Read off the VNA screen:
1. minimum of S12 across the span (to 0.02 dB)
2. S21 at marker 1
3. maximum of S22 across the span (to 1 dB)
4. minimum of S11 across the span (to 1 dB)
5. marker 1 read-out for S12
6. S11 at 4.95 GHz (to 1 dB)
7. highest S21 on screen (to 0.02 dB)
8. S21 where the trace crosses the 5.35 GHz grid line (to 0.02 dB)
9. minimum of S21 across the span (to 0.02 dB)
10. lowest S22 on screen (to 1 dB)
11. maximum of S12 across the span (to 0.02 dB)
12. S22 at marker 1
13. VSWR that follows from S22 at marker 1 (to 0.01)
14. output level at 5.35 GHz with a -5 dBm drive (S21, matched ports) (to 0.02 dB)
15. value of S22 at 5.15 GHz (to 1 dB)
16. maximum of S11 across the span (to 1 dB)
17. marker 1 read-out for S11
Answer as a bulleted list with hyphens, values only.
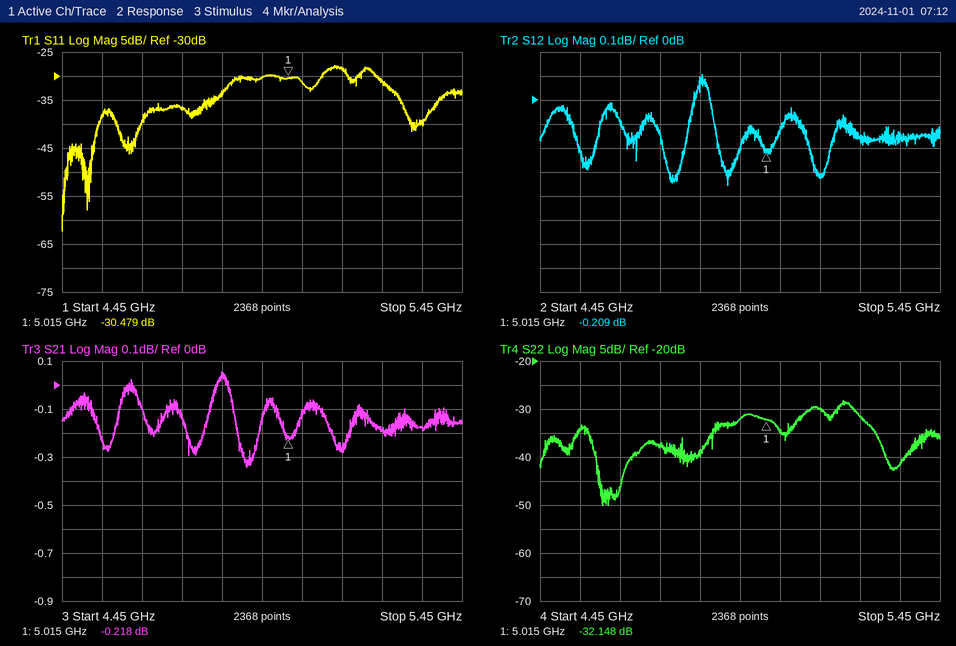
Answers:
- -0.36 dB
- -0.218 dB
- -28 dB
- -62 dB
- -0.209 dB
- -30 dB
- 0.06 dB
- -0.18 dB
- -0.34 dB
- -50 dB
- 0.10 dB
- -32.148 dB
- 1.05
- -5.18 dBm
- -30 dB
- -28 dB
- -30.479 dB
